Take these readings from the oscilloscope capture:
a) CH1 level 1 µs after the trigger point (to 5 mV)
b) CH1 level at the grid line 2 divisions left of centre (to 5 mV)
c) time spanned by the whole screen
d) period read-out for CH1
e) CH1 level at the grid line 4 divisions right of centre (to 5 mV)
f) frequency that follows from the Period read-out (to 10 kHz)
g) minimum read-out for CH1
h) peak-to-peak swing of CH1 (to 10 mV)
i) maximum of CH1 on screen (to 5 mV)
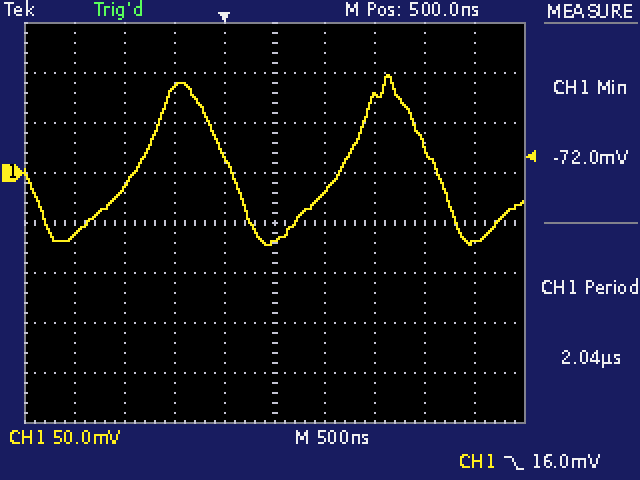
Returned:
-20 mV
85 mV
5 µs
2.04 µs
-70 mV
490 kHz
-72.0 mV
170 mV
100 mV
